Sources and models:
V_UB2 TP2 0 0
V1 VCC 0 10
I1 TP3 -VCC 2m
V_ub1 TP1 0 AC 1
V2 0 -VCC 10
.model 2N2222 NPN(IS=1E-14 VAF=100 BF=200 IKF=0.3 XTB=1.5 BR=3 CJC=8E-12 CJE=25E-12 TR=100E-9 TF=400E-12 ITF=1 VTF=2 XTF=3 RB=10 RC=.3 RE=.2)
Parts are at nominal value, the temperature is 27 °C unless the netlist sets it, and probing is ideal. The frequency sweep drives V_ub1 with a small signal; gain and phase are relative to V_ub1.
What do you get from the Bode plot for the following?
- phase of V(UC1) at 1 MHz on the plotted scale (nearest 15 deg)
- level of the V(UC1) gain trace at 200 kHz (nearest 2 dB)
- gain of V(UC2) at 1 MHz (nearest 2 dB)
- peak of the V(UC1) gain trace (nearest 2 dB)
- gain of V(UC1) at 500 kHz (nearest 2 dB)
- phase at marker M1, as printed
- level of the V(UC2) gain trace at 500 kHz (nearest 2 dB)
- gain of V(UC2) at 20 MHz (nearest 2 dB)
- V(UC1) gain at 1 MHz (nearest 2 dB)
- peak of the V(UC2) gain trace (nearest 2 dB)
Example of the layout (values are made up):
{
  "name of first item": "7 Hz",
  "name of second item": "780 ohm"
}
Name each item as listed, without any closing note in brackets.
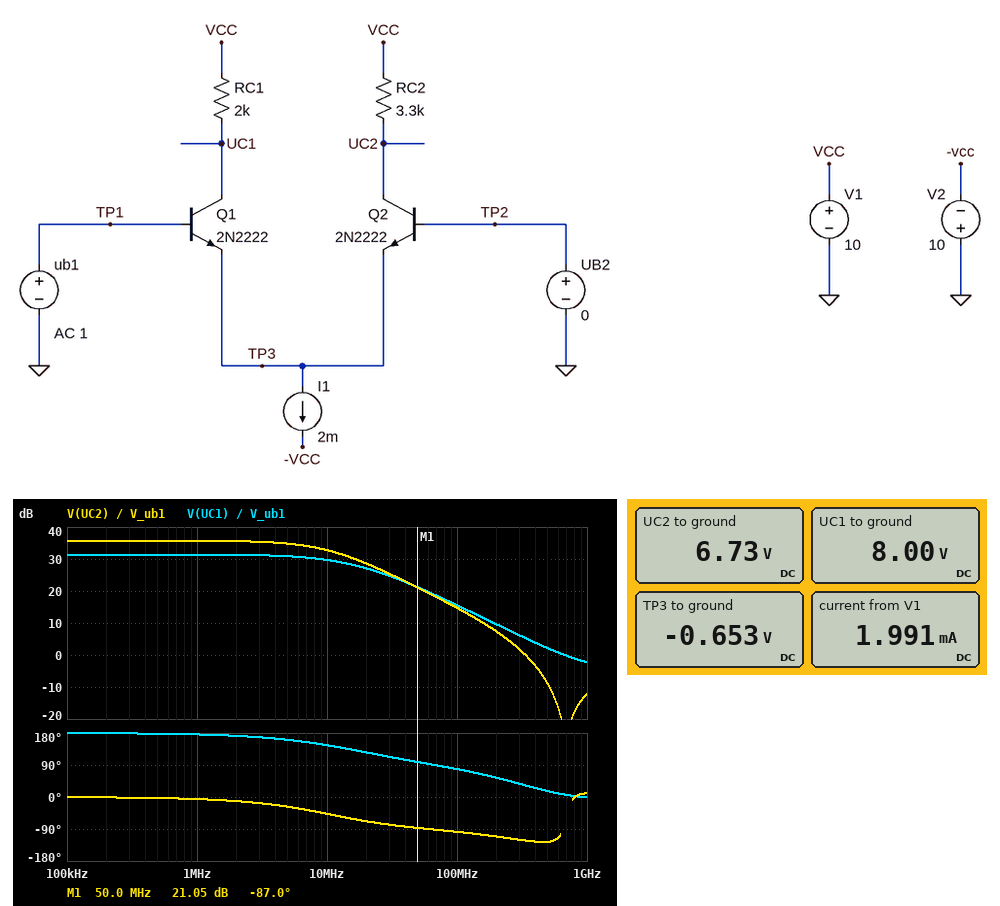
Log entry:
{
  "phase of V(UC1) at 1 MHz on the plotted scale": "180 deg",
  "level of the V(UC1) gain trace at 200 kHz": "32 dB",
  "gain of V(UC2) at 1 MHz": "36 dB",
  "peak of the V(UC1) gain trace": "32 dB",
  "gain of V(UC1) at 500 kHz": "32 dB",
  "phase at marker M1, as printed": "-87.0 deg",
  "level of the V(UC2) gain trace at 500 kHz": "36 dB",
  "gain of V(UC2) at 20 MHz": "28 dB",
  "V(UC1) gain at 1 MHz": "32 dB",
  "peak of the V(UC2) gain trace": "36 dB"
}
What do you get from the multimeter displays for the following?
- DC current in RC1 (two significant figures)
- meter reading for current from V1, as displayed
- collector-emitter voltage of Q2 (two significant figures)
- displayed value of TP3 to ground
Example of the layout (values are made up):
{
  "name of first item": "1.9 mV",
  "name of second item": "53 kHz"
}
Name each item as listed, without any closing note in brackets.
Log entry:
{
  "DC current in RC1": "1.0 mA",
  "meter reading for current from V1, as displayed": "1.991 mA",
  "collector-emitter voltage of Q2": "7.4 V",
  "displayed value of TP3 to ground": "-0.653 V"
}
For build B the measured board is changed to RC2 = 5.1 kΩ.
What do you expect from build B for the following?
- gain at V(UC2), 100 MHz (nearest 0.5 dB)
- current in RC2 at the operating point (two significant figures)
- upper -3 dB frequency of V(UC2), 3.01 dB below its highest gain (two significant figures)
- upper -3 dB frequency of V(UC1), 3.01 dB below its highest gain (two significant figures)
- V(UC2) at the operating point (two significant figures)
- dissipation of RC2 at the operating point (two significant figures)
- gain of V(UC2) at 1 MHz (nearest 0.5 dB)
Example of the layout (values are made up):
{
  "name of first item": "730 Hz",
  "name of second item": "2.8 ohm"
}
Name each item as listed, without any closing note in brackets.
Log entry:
{
  "gain at V(UC2), 100 MHz": "14.0 dB",
  "current in RC2 at the operating point": "980 µA",
  "upper -3 dB frequency of V(UC2), 3.01 dB below its highest gain": "6.3 MHz",
  "upper -3 dB frequency of V(UC1), 3.01 dB below its highest gain": "14 MHz",
  "V(UC2) at the operating point": "5.0 V",
  "dissipation of RC2 at the operating point": "4.9 mW",
  "gain of V(UC2) at 1 MHz": "39.5 dB"
}
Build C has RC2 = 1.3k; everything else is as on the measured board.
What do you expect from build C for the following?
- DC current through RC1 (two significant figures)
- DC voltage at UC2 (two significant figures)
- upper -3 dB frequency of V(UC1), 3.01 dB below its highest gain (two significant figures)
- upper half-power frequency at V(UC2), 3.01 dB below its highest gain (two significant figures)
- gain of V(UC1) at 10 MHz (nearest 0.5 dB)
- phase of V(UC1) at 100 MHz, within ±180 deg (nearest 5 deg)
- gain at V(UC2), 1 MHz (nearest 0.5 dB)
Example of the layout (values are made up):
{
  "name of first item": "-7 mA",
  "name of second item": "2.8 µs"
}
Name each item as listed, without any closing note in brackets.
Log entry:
{
  "DC current through RC1": "990 µA",
  "DC voltage at UC2": "8.7 V",
  "upper -3 dB frequency of V(UC1), 3.01 dB below its highest gain": "17 MHz",
  "upper half-power frequency at V(UC2), 3.01 dB below its highest gain": "23 MHz",
  "gain of V(UC1) at 10 MHz": "30.0 dB",
  "phase of V(UC1) at 100 MHz, within ±180 deg": "75 deg",
  "gain at V(UC2), 1 MHz": "27.5 dB"
}
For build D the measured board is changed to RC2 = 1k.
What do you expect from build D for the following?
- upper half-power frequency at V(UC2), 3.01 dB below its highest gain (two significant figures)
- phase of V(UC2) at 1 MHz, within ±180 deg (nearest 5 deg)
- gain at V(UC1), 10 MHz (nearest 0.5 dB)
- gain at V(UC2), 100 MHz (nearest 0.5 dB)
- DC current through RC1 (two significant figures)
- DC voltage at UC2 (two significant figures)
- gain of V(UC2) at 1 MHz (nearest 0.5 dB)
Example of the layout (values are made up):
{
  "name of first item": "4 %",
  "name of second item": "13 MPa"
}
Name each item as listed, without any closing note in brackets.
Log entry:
{
  "upper half-power frequency at V(UC2), 3.01 dB below its highest gain": "29 MHz",
  "phase of V(UC2) at 1 MHz, within ±180 deg": "0 deg",
  "gain at V(UC1), 10 MHz": "30.5 dB",
  "gain at V(UC2), 100 MHz": "15.0 dB",
  "DC current through RC1": "990 µA",
  "DC voltage at UC2": "9.0 V",
  "gain of V(UC2) at 1 MHz": "25.5 dB"
}
